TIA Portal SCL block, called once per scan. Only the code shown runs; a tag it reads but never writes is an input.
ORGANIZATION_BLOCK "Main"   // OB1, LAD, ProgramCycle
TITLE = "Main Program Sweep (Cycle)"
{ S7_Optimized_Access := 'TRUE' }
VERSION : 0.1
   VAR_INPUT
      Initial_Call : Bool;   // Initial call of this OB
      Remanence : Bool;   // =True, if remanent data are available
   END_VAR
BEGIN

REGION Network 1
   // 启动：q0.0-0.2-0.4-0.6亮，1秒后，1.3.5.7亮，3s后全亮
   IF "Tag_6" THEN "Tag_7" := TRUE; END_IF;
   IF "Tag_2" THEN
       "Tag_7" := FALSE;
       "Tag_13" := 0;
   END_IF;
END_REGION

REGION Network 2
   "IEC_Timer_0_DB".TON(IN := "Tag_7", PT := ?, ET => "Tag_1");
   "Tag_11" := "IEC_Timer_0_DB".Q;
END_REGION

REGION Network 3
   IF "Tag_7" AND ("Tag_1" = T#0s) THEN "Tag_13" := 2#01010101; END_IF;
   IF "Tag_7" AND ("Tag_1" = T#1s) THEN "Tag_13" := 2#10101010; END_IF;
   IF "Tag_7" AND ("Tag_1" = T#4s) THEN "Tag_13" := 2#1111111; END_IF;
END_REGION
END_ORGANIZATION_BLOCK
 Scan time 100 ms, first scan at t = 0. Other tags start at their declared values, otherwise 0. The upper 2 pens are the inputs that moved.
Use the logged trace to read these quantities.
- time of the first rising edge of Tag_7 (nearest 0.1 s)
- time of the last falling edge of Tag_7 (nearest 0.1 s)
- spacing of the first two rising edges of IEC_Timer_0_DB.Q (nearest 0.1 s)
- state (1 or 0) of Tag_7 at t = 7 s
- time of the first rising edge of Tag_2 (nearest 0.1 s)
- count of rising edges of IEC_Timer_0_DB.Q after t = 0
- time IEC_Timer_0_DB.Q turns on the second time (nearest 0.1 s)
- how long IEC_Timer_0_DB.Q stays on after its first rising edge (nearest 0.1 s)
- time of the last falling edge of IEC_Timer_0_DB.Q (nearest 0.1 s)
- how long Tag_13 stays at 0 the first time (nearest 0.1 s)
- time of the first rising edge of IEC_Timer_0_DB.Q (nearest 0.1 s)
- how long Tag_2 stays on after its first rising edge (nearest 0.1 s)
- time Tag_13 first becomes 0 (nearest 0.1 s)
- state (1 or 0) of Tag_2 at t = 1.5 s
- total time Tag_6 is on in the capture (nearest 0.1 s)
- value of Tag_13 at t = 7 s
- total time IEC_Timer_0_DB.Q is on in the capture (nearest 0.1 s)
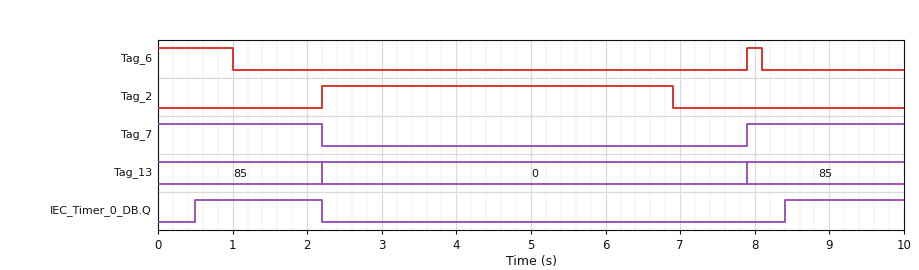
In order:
7.9 s
2.2 s
7.9 s
0
2.2 s
2
8.4 s
1.7 s
2.2 s
5.7 s
0.5 s
4.7 s
2.2 s
0
1.2 s
0
3.3 s
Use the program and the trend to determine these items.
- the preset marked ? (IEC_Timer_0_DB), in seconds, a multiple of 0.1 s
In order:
0.5 s
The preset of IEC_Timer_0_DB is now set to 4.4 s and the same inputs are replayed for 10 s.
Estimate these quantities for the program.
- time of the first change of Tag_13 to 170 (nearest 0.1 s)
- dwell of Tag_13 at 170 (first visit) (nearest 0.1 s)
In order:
1.0 s
1.2 s
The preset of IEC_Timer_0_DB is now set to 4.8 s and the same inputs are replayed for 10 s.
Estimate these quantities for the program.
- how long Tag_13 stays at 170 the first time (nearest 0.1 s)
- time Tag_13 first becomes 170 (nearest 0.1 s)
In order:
1.2 s
1.0 s
